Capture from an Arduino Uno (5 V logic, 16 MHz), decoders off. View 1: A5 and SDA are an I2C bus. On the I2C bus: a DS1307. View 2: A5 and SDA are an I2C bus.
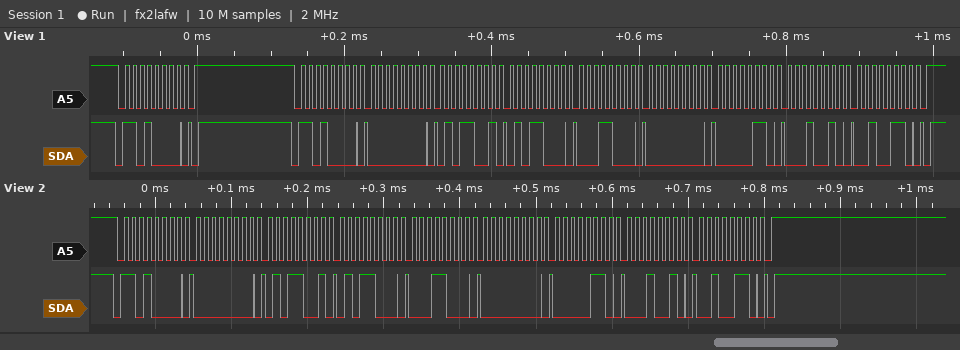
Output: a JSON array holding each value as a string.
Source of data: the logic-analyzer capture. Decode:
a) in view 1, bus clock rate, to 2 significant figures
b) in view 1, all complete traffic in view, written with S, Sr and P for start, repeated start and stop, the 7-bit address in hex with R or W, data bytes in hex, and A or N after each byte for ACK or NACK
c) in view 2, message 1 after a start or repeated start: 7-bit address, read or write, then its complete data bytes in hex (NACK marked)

["100 kHz", "S 68W A P S 68W A 00 A 59 A 58 A 18 A 00 A 06 A 12 A 26 A P", "0x68 write: 00 59 58 18 00 06 12 26"]
